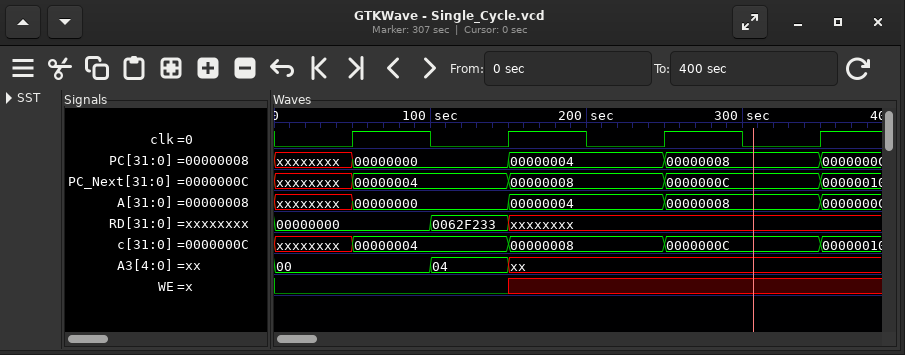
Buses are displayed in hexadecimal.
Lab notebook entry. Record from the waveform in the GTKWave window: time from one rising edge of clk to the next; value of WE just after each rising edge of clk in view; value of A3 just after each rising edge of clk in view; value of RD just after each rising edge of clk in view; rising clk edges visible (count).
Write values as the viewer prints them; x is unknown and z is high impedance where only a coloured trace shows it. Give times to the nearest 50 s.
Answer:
100 s
0 x x x
00, xx, xx, xx
00000000, xxxxxxxx, xxxxxxxx, xxxxxxxx
4
